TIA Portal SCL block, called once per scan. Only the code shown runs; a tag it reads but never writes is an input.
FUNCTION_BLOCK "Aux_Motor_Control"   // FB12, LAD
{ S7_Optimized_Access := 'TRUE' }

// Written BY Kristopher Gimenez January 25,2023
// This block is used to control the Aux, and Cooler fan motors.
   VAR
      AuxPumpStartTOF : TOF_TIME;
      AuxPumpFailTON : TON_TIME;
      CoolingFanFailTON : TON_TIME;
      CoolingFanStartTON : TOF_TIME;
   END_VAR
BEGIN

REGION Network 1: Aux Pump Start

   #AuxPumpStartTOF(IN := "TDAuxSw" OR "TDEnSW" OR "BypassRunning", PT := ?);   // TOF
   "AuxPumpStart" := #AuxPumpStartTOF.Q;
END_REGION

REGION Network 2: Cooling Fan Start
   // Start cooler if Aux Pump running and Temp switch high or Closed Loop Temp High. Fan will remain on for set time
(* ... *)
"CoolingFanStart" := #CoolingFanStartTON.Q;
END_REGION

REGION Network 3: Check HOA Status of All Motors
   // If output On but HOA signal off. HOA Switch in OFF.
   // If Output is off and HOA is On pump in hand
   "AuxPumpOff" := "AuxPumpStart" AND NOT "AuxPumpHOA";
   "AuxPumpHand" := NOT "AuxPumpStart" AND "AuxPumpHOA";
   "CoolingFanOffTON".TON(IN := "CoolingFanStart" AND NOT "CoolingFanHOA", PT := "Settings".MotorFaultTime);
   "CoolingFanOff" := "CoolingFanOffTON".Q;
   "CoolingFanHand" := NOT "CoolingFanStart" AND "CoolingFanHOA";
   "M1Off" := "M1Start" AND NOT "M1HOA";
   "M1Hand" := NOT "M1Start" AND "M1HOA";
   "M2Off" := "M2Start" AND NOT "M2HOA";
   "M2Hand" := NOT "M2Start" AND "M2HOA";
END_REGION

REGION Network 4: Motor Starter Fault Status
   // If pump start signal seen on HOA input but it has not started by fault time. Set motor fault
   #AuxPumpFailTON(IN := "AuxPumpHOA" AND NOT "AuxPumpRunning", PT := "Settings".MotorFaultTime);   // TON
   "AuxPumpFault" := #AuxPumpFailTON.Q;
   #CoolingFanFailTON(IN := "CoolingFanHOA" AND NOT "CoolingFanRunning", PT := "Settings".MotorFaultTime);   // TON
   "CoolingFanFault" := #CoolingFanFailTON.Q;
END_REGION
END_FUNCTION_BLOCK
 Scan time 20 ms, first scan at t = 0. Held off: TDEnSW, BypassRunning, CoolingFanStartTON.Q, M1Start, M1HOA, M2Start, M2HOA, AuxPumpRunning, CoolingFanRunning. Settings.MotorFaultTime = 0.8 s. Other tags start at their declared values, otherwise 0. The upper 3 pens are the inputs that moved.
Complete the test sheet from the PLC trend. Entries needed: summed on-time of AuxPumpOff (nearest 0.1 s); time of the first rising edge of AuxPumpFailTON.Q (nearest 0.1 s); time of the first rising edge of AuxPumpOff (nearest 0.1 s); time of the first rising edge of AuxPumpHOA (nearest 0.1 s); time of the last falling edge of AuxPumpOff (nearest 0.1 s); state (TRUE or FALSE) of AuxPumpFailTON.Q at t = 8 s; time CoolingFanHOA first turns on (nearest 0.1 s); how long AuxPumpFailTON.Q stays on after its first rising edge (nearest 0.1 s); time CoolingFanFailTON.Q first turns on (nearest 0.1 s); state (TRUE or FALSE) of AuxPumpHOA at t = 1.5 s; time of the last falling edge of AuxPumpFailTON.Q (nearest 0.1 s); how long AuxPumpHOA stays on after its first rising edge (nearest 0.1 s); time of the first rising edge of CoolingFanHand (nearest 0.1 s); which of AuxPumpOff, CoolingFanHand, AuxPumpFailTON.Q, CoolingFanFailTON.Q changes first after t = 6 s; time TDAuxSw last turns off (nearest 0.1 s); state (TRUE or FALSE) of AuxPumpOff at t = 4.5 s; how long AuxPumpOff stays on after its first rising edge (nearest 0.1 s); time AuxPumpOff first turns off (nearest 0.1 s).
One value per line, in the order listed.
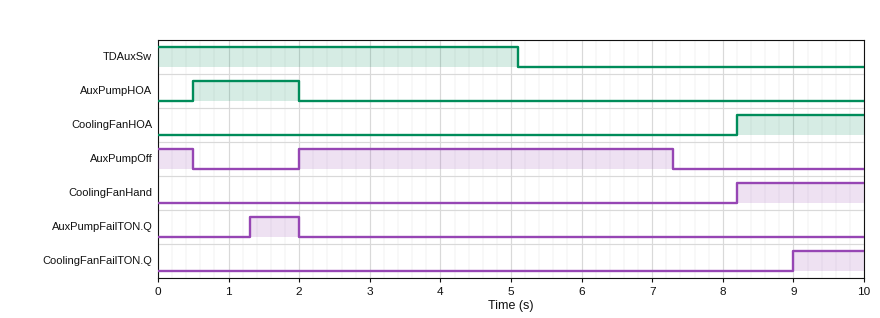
5.8 s
1.3 s
2.0 s
0.5 s
7.3 s
FALSE
8.2 s
0.7 s
9.0 s
TRUE
2.0 s
1.5 s
8.2 s
AuxPumpOff
5.1 s
TRUE
5.3 s
0.5 s
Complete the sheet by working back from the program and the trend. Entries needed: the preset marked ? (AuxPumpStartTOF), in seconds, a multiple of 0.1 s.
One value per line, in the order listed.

2.2 s
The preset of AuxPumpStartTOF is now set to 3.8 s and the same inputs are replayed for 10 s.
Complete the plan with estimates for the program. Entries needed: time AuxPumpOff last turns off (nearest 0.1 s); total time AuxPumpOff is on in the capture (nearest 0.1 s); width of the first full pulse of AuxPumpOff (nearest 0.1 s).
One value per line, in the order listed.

8.9 s
7.4 s
6.9 s
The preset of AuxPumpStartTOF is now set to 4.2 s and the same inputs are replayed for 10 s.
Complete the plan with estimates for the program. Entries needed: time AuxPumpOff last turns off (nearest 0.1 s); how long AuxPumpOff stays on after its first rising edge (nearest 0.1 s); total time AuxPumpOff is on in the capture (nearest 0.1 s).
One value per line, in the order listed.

9.3 s
7.3 s
7.8 s
